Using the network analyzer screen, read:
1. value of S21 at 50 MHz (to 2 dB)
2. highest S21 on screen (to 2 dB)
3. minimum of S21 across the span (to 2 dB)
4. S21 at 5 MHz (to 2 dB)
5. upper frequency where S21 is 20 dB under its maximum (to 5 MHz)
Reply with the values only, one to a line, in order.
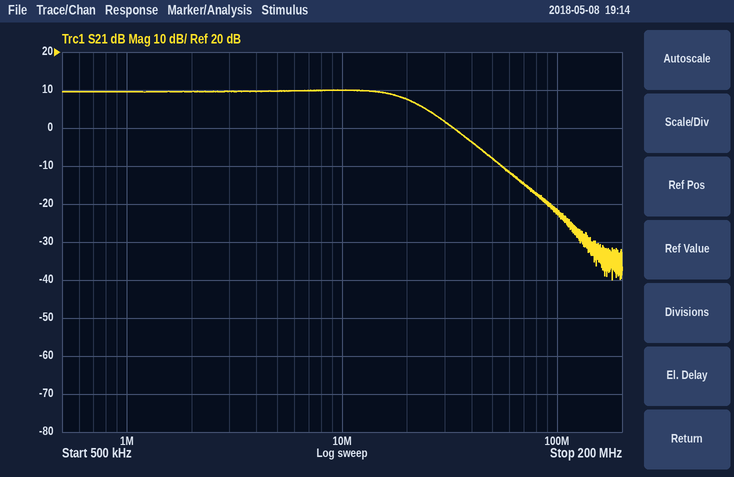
-8 dB
10 dB
-40 dB
10 dB
55 MHz
